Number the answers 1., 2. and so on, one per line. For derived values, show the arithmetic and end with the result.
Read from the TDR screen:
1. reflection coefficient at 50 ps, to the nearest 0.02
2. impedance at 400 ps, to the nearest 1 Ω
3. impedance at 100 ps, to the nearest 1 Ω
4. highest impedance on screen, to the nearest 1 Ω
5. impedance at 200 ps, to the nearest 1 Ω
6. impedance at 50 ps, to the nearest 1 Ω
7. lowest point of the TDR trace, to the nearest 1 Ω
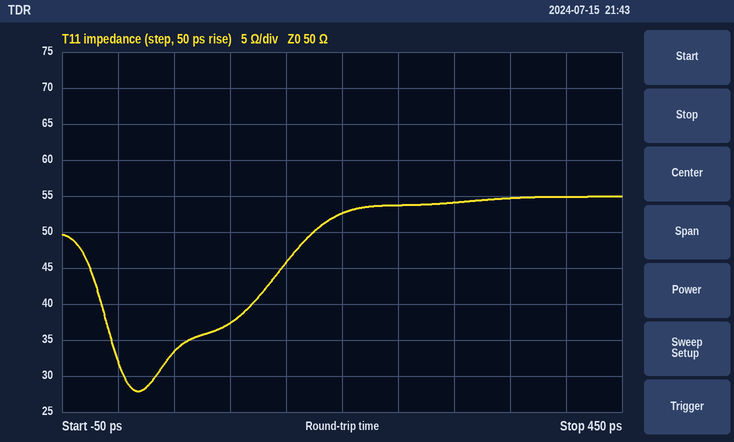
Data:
1. (33 − 50)/(33 + 50) ≈ -0.20
2. 55 Ω
3. 37 Ω
4. 55 Ω
5. 53 Ω
6. 33 Ω
7. 28 Ω
